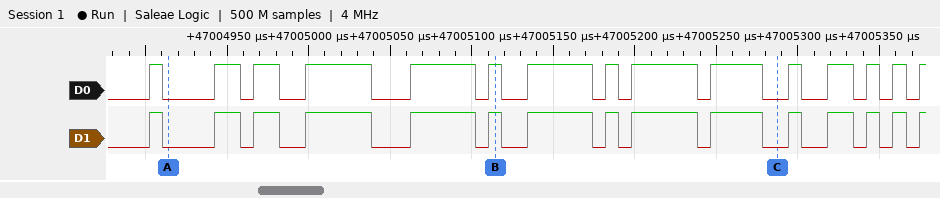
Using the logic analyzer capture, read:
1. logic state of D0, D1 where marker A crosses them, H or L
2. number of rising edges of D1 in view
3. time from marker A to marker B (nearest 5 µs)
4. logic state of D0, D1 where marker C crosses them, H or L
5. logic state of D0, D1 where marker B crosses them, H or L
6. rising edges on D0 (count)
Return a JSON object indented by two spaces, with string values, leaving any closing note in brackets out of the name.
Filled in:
{
  "logic state of D0, D1 where marker A crosses them, H or L": "D0=L, D1=L",
  "number of rising edges of D1 in view": "15",
  "time from marker A to marker B": "200 µs",
  "logic state of D0, D1 where marker C crosses them, H or L": "D0=L, D1=L",
  "logic state of D0, D1 where marker B crosses them, H or L": "D0=H, D1=H",
  "rising edges on D0": "15"
}
